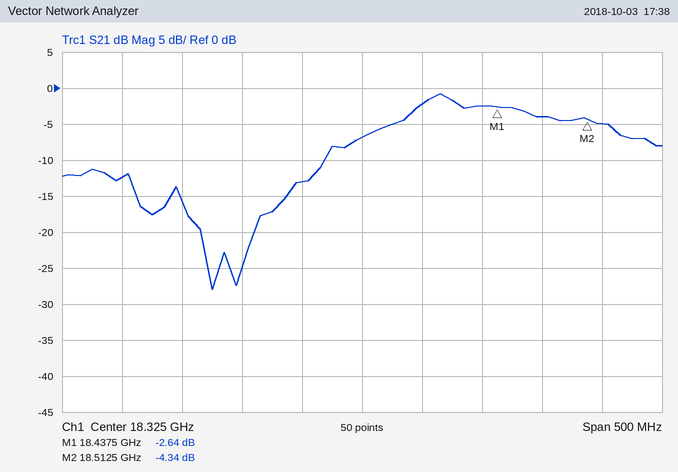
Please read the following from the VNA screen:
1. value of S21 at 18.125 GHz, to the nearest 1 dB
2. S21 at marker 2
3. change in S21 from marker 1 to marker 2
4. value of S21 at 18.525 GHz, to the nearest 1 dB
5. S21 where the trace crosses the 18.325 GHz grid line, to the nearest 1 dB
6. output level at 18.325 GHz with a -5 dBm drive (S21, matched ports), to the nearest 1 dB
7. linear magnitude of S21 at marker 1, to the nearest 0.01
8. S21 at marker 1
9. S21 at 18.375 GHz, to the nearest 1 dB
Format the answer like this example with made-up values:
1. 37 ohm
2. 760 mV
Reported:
1. -12 dB
2. -4.34 dB
3. -1.70 dB
4. -5 dB
5. -7 dB
6. -12 dBm
7. 0.74
8. -2.64 dB
9. -2 dB
